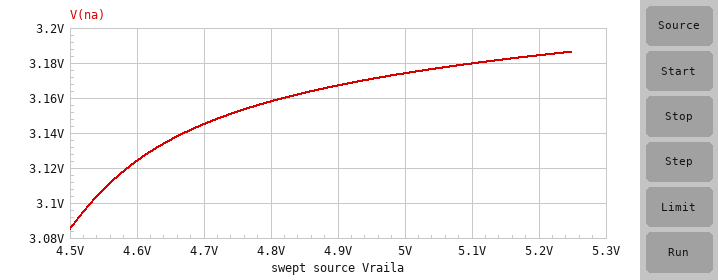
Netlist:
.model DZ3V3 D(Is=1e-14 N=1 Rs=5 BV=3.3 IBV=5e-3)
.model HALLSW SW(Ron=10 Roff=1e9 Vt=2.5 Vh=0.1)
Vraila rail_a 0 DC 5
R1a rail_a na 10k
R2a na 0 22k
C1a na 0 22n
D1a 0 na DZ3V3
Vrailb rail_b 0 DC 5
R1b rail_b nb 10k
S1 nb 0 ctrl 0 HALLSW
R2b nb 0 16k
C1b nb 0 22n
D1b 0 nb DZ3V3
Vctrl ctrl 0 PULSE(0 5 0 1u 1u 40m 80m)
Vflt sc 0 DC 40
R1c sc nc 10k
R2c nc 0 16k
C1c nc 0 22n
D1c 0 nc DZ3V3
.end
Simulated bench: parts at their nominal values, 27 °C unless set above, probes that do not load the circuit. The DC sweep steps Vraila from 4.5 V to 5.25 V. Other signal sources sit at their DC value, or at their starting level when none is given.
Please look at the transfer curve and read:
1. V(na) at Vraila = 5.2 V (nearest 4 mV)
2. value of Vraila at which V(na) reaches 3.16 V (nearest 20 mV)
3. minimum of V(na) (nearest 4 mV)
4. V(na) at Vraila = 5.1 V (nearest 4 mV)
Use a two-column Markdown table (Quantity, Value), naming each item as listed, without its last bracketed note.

| Quantity | Value |
|---|---|
| V(na) at Vraila = 5.2 V | 3.184 V |
| value of Vraila at which V(na) reaches 3.16 V | 4.82 V |
| minimum of V(na) | 3.084 V |
| V(na) at Vraila = 5.1 V | 3.180 V |
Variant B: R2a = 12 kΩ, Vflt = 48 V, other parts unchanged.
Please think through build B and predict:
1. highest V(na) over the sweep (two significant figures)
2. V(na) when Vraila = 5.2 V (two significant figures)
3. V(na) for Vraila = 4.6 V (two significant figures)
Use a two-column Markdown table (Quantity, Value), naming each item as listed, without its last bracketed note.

| Quantity | Value |
|---|---|
| highest V(na) over the sweep | 2.9 V |
| V(na) when Vraila = 5.2 V | 2.8 V |
| V(na) for Vraila = 4.6 V | 2.5 V |
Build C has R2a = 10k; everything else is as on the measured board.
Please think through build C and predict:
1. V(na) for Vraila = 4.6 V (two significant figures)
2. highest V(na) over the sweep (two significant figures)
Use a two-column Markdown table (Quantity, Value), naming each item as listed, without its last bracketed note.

| Quantity | Value |
|---|---|
| V(na) for Vraila = 4.6 V | 2.3 V |
| highest V(na) over the sweep | 2.6 V |
